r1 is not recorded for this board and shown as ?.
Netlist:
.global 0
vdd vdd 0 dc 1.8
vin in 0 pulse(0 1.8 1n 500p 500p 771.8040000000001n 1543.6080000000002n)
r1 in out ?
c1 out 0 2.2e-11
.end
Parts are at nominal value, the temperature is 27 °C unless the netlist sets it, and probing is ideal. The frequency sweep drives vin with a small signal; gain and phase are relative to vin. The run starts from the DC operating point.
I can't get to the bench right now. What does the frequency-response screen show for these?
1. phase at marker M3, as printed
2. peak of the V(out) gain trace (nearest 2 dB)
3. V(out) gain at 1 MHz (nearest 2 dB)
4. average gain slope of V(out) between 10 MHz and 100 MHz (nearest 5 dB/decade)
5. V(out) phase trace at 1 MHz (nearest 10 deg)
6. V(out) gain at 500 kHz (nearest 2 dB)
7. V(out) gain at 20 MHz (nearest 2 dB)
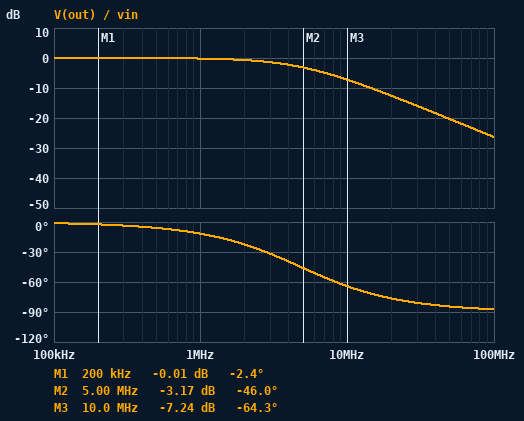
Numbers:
-64.3 deg
0 dB
0 dB
-20 dB/decade
-10 deg
0 dB
-12 dB
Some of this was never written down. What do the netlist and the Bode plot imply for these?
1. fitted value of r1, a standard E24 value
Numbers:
1.5 kΩ
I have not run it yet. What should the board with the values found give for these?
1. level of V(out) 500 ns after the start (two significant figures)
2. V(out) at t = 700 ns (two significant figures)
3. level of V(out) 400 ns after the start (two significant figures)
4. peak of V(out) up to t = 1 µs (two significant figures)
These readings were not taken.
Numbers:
1.8 V
1.8 V
1.8 V
1.8 V
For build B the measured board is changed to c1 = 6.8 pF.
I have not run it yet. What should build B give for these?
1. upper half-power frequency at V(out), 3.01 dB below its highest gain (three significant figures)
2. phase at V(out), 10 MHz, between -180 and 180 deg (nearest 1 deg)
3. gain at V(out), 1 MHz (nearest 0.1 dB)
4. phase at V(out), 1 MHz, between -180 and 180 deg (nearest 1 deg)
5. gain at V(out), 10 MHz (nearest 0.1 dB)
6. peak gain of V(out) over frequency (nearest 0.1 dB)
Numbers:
15.6 MHz
-33 deg
0 dB
-4 deg
-1.5 dB
0 dB
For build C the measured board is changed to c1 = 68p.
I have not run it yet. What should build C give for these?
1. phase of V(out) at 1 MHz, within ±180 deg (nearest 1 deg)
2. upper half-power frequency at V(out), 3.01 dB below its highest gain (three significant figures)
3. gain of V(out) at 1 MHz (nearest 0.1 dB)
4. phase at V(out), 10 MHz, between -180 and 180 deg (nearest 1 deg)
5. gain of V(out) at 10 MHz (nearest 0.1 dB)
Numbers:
-33 deg
1.56 MHz
-1.5 dB
-81 deg
-16.2 dB
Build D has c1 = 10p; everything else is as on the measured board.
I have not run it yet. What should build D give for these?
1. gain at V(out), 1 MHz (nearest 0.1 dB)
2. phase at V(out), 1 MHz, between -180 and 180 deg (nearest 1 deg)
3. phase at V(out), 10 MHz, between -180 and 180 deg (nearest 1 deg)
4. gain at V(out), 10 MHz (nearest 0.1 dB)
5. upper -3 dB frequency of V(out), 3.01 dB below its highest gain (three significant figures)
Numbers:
0 dB
-5 deg
-43 deg
-2.8 dB
10.6 MHz
